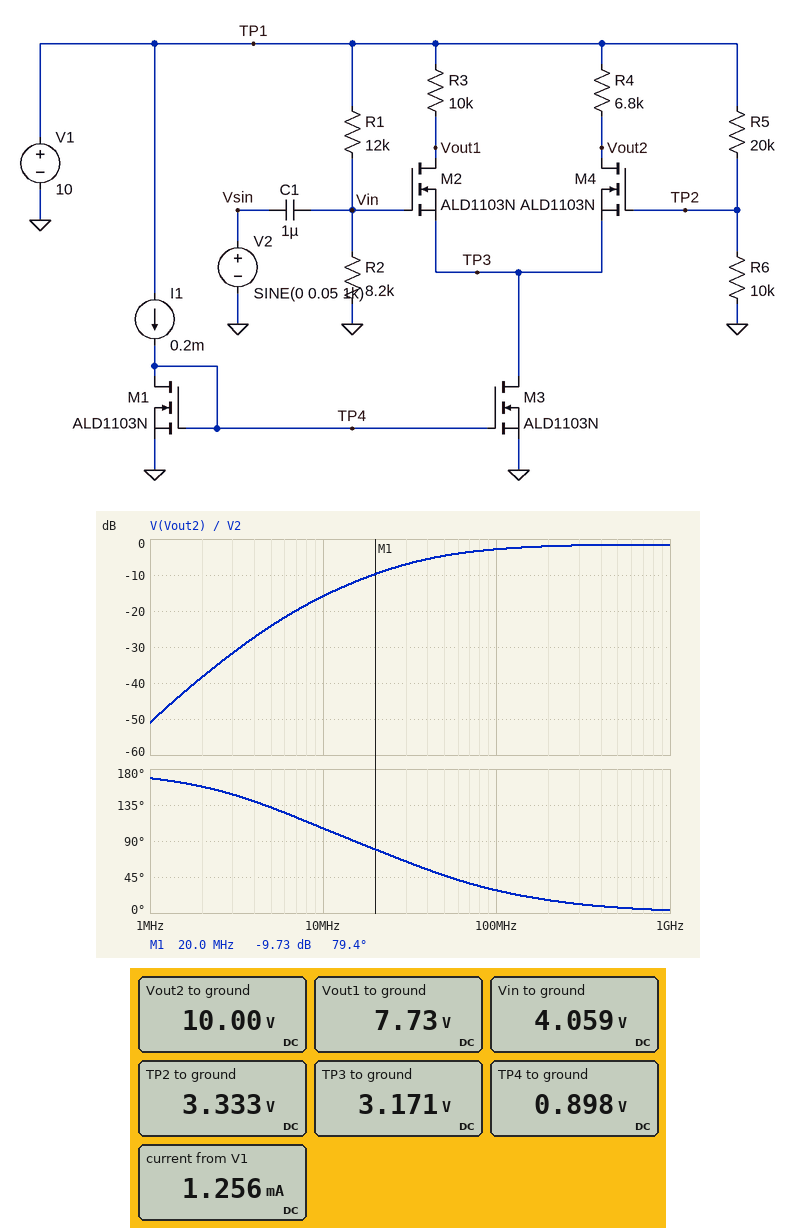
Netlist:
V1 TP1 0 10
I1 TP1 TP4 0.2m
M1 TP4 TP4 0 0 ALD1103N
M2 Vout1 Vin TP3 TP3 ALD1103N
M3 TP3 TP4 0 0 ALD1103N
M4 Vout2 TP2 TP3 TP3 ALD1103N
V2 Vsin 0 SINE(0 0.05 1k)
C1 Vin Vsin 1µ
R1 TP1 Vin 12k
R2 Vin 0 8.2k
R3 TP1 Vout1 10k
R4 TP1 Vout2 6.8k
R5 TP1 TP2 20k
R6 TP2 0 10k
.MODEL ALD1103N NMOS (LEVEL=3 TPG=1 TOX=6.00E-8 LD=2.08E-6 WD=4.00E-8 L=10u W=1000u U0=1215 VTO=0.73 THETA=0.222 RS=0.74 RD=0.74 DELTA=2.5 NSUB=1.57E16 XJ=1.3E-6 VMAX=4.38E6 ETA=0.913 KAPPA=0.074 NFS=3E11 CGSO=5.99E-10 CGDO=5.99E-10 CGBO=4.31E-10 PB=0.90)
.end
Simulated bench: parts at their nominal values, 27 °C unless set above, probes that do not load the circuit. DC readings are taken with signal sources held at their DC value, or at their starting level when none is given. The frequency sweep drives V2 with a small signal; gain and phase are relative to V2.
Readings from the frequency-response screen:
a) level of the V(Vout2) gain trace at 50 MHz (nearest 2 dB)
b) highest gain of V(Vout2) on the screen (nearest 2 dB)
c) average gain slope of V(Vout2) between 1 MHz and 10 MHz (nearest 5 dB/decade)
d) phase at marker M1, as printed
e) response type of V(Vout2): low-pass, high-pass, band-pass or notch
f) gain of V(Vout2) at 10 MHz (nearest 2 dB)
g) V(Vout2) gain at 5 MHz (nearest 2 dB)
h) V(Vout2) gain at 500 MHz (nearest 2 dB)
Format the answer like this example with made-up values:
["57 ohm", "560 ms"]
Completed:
["-4 dB", "-2 dB", "35 dB/decade", "79.4 deg", "high-pass", "-16 dB", "-24 dB", "-2 dB"]
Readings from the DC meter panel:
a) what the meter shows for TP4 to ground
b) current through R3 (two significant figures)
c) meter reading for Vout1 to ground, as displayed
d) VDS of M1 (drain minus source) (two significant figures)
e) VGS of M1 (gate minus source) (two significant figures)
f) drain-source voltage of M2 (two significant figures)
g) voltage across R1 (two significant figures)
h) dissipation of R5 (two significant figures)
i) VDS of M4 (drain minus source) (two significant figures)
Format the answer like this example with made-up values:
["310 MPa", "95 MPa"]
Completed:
["0.898 V", "230 µA", "7.73 V", "900 mV", "900 mV", "4.6 V", "5.9 V", "2.2 mW", "6.8 V"]
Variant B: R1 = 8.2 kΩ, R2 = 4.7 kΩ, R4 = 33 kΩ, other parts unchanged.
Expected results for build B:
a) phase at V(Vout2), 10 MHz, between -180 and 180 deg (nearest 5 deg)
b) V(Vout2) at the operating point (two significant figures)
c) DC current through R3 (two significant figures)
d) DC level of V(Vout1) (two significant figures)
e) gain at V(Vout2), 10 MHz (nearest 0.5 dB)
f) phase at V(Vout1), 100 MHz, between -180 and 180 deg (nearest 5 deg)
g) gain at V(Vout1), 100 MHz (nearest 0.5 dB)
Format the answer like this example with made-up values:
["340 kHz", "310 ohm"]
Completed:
["10 deg", "9.9 V", "220 µA", "7.8 V", "-19.5 dB", "60 deg", "1.5 dB"]
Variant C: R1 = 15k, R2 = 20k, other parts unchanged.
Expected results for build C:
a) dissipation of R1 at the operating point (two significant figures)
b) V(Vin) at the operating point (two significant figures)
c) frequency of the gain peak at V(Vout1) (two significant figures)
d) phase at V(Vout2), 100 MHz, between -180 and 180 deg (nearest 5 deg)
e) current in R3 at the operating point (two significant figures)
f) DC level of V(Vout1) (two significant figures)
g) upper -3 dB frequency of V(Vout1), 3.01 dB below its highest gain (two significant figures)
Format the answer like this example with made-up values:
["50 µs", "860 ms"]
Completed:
["1.2 mW", "5.7 V", "28 MHz", "25 deg", "250 µA", "7.5 V", "120 MHz"]
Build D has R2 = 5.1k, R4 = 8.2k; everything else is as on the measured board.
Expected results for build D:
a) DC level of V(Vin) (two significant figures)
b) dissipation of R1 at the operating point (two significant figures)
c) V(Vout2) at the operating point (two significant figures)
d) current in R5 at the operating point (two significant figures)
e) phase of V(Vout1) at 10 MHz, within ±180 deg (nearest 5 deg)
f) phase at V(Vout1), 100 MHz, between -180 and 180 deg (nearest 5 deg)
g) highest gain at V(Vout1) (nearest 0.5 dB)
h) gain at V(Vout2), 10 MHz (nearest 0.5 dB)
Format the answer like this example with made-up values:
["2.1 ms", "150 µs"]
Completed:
["3.0 V", "4.1 mW", "8.2 V", "330 µA", "90 deg", "15 deg", "0 dB", "3.5 dB"]
